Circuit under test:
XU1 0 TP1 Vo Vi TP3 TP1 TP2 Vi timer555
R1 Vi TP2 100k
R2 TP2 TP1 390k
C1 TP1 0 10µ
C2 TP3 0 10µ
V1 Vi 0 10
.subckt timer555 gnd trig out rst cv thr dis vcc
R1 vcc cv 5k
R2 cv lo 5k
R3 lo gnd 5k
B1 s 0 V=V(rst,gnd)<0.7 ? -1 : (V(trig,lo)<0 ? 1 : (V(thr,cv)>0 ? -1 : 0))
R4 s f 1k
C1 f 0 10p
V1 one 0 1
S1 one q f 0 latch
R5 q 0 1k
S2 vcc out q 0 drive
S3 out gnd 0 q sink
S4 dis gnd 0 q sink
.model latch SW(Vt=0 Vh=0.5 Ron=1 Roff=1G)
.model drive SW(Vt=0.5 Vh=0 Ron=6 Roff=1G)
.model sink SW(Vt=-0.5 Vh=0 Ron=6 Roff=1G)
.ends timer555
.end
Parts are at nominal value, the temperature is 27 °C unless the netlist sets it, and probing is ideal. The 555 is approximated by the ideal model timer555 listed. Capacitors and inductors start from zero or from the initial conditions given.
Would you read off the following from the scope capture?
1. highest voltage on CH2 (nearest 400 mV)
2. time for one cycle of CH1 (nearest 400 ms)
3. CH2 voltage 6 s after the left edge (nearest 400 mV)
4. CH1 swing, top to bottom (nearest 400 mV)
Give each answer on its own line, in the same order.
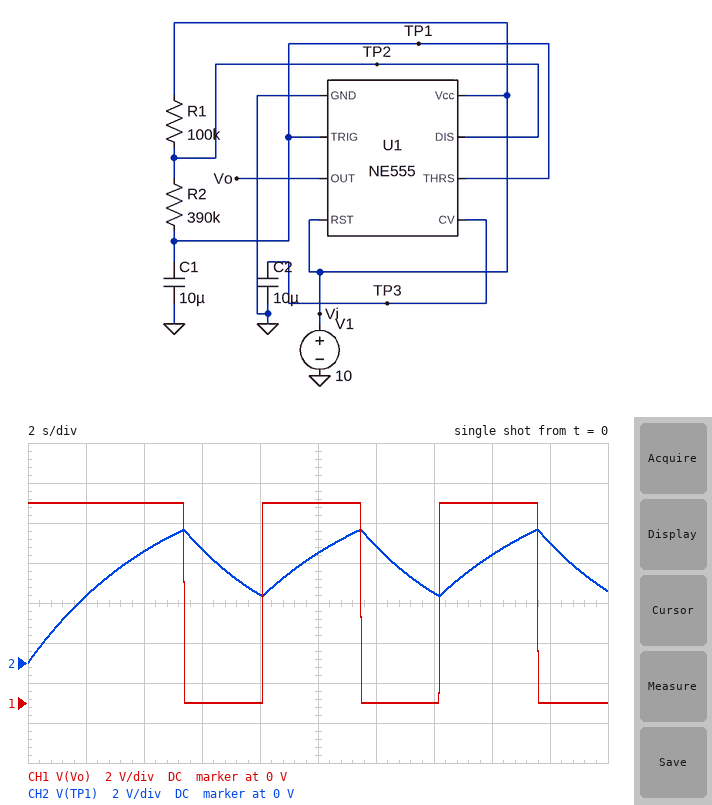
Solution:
6.8 V
6.0 s
5.6 V
10.0 V
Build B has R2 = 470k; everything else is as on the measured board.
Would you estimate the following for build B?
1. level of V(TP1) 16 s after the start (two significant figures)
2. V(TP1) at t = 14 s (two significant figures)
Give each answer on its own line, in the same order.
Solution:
3.9 V
6.0 V
